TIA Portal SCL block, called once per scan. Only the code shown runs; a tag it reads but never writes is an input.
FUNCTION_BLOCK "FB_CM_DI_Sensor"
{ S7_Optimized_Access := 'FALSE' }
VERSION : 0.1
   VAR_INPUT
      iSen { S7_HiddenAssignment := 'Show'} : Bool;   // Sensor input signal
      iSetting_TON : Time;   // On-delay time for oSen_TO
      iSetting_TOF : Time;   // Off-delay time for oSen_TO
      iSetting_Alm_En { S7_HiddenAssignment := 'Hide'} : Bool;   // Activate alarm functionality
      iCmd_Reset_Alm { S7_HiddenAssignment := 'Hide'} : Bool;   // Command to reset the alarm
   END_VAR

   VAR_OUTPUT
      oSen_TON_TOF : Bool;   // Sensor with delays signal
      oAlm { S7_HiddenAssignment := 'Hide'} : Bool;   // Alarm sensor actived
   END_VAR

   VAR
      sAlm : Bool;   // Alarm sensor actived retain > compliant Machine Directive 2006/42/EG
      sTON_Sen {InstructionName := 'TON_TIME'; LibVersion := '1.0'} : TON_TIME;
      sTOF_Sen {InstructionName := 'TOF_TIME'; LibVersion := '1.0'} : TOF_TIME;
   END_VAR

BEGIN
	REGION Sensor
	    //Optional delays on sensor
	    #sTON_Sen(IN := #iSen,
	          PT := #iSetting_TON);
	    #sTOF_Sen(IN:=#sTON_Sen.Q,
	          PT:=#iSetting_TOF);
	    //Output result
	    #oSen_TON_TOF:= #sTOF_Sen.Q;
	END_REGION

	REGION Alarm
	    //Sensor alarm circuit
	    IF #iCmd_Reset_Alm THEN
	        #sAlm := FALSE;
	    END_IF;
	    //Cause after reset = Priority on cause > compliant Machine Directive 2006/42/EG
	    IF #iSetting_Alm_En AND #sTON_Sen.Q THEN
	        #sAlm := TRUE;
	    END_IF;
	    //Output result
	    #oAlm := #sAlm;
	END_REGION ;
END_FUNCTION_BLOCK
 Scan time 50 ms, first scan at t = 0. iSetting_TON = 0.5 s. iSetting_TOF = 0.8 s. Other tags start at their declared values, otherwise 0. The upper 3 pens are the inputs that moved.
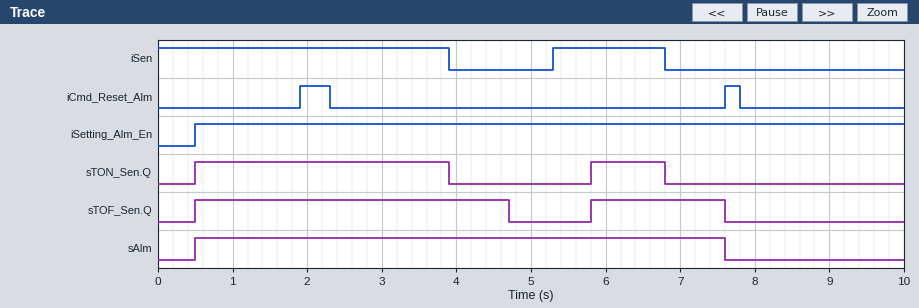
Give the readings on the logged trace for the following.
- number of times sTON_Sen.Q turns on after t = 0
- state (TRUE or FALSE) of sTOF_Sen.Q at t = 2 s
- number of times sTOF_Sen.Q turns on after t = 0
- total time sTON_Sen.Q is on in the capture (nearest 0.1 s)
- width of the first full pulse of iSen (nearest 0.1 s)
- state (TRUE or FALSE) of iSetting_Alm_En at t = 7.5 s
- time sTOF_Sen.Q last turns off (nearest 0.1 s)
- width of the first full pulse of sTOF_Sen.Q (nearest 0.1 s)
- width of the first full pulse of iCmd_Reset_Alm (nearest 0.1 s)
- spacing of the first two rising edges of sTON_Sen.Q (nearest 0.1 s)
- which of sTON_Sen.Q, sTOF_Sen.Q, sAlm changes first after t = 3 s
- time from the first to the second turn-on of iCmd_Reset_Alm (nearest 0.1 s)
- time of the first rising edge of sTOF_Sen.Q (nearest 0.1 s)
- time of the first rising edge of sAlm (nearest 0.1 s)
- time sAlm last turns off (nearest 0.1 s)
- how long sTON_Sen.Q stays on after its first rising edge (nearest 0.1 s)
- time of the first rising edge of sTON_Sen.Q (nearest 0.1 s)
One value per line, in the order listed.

2
TRUE
2
4.4 s
1.5 s
TRUE
7.6 s
4.2 s
0.4 s
5.3 s
sTON_Sen.Q
5.7 s
0.5 s
0.5 s
7.6 s
3.4 s
0.5 s
